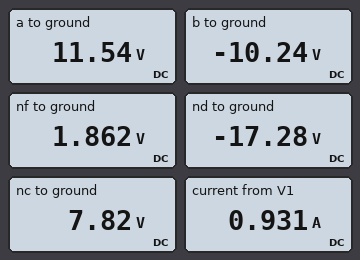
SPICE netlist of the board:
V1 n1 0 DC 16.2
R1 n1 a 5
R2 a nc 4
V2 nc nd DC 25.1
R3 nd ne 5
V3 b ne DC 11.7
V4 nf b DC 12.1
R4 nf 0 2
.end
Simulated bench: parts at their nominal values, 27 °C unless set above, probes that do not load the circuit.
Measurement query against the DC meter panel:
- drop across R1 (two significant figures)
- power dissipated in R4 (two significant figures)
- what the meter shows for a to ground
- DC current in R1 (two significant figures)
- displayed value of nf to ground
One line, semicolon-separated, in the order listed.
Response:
4.7 V; 1.7 W; 11.54 V; 930 mA; 1.862 V
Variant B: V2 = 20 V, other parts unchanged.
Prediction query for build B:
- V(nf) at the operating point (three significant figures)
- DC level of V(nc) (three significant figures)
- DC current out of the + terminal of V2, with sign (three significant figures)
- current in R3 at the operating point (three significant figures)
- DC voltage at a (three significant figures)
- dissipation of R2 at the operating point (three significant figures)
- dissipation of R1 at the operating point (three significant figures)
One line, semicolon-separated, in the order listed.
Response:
2.50 V; 4.95 V; -1.25 A; 1.25 A; 9.95 V; 6.25 W; 7.81 W
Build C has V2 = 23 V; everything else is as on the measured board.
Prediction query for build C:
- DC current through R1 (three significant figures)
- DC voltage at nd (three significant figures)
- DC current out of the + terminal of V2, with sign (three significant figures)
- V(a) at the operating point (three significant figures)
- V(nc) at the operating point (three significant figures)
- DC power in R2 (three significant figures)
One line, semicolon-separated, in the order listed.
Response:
1.06 A; -16.4 V; -1.06 A; 10.9 V; 6.64 V; 4.52 W
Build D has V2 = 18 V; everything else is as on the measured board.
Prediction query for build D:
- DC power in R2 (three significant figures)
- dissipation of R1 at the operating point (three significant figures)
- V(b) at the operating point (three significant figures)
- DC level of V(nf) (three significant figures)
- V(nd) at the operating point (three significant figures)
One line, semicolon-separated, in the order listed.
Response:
7.56 W; 9.45 W; -9.35 V; 2.75 V; -14.2 V
